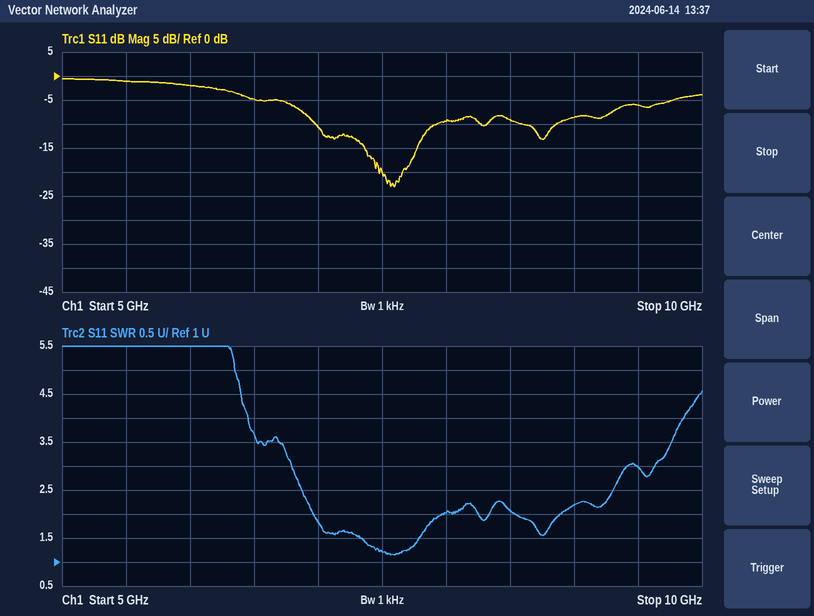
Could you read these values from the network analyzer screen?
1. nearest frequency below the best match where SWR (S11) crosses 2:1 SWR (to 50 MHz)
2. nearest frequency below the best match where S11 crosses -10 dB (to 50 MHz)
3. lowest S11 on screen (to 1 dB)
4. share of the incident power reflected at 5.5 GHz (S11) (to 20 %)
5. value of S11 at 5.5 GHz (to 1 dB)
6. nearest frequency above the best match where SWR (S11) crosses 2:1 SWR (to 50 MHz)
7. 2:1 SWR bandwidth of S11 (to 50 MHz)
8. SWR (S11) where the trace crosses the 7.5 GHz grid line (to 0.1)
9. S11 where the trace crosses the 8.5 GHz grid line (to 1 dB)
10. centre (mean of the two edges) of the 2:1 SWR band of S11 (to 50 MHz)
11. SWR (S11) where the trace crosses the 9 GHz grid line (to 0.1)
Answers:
6.95 GHz
7.00 GHz
-23 dB
80 %
-1 dB
7.95 GHz
1.00 GHz
1.2
-9 dB
7.45 GHz
2.2
